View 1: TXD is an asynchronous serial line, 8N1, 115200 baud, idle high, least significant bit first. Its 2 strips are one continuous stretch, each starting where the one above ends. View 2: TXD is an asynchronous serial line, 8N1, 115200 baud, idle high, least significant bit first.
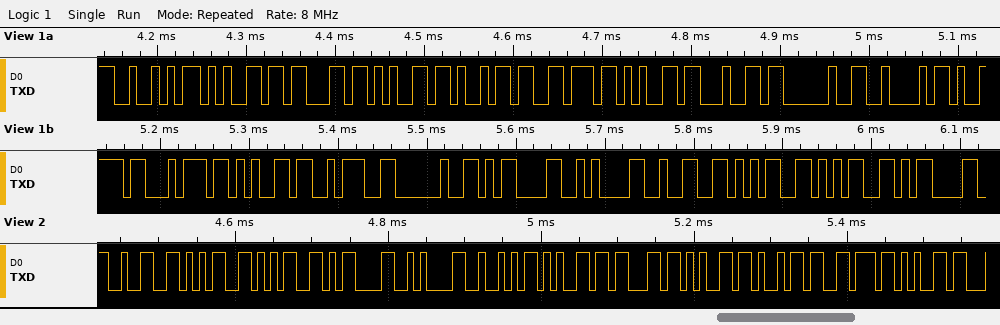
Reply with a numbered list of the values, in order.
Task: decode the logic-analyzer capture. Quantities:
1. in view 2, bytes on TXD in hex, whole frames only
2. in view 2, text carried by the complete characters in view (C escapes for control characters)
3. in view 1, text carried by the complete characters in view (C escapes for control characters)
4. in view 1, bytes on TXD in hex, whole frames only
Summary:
1. 32 35 35 0D 0A 52 65 63 65 69 76 65
2. "255\r\nReceive"
3. "Received Byte: \r\n255\r"
4. 52 65 63 65 69 76 65 64 20 42 79 74 65 3A 20 0D 0A 32 35 35 0D
